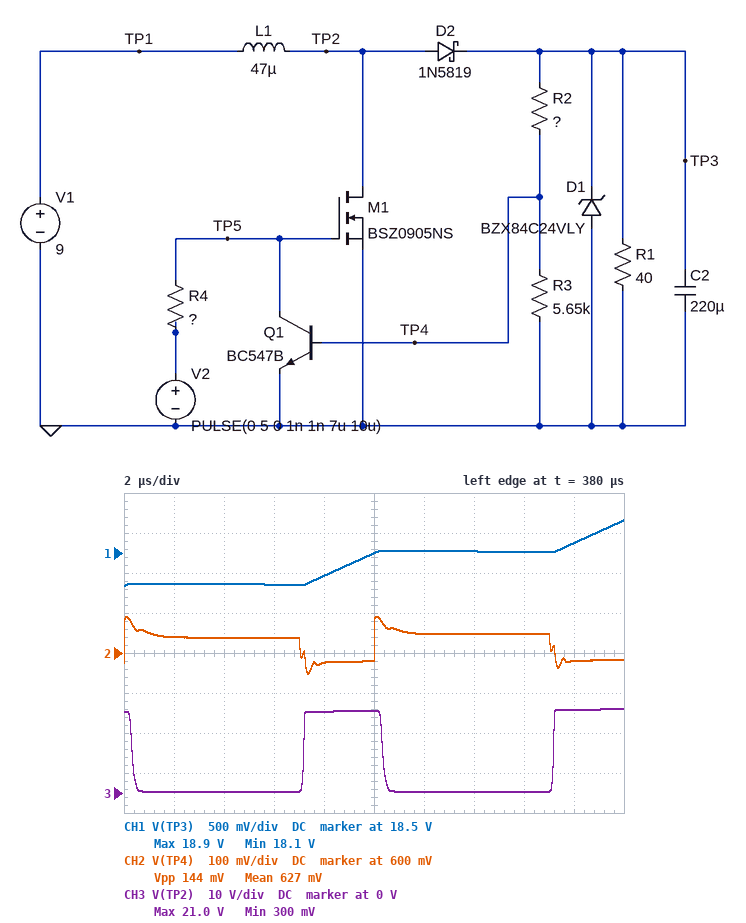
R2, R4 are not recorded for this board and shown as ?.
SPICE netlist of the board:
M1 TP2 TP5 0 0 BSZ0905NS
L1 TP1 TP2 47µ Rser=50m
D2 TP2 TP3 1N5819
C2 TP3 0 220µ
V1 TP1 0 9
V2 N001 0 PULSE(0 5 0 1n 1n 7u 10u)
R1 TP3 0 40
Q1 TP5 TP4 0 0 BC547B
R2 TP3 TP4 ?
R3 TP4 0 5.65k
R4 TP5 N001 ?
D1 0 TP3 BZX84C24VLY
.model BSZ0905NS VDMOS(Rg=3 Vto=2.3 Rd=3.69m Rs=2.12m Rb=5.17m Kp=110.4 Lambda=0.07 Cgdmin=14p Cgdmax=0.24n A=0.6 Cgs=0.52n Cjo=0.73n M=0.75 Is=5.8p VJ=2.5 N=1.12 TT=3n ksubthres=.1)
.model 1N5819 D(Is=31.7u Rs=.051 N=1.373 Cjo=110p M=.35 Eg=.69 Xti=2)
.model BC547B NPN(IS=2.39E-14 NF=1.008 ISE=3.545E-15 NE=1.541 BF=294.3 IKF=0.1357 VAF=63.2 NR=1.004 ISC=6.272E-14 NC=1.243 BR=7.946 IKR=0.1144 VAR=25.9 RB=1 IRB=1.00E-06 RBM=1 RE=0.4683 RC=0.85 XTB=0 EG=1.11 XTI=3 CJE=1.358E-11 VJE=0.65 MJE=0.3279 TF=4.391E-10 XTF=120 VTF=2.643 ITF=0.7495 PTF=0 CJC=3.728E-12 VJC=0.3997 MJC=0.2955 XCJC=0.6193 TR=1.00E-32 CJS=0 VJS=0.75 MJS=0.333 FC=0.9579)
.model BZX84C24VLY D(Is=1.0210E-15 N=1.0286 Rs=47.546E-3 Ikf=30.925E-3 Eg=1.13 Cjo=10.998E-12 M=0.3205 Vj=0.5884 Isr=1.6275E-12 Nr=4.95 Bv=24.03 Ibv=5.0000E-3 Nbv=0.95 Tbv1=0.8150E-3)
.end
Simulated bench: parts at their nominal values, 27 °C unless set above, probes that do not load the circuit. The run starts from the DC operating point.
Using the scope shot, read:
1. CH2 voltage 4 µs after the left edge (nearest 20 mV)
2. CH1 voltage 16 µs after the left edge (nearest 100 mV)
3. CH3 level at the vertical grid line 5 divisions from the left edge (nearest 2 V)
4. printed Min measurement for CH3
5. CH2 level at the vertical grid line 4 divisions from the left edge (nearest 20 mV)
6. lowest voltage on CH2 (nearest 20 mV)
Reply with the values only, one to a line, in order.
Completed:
640 mV
18.5 V
20 V
300 mV
580 mV
540 mV
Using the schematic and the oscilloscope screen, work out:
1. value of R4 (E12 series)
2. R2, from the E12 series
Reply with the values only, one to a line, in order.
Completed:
270 Ω
150 kΩ
